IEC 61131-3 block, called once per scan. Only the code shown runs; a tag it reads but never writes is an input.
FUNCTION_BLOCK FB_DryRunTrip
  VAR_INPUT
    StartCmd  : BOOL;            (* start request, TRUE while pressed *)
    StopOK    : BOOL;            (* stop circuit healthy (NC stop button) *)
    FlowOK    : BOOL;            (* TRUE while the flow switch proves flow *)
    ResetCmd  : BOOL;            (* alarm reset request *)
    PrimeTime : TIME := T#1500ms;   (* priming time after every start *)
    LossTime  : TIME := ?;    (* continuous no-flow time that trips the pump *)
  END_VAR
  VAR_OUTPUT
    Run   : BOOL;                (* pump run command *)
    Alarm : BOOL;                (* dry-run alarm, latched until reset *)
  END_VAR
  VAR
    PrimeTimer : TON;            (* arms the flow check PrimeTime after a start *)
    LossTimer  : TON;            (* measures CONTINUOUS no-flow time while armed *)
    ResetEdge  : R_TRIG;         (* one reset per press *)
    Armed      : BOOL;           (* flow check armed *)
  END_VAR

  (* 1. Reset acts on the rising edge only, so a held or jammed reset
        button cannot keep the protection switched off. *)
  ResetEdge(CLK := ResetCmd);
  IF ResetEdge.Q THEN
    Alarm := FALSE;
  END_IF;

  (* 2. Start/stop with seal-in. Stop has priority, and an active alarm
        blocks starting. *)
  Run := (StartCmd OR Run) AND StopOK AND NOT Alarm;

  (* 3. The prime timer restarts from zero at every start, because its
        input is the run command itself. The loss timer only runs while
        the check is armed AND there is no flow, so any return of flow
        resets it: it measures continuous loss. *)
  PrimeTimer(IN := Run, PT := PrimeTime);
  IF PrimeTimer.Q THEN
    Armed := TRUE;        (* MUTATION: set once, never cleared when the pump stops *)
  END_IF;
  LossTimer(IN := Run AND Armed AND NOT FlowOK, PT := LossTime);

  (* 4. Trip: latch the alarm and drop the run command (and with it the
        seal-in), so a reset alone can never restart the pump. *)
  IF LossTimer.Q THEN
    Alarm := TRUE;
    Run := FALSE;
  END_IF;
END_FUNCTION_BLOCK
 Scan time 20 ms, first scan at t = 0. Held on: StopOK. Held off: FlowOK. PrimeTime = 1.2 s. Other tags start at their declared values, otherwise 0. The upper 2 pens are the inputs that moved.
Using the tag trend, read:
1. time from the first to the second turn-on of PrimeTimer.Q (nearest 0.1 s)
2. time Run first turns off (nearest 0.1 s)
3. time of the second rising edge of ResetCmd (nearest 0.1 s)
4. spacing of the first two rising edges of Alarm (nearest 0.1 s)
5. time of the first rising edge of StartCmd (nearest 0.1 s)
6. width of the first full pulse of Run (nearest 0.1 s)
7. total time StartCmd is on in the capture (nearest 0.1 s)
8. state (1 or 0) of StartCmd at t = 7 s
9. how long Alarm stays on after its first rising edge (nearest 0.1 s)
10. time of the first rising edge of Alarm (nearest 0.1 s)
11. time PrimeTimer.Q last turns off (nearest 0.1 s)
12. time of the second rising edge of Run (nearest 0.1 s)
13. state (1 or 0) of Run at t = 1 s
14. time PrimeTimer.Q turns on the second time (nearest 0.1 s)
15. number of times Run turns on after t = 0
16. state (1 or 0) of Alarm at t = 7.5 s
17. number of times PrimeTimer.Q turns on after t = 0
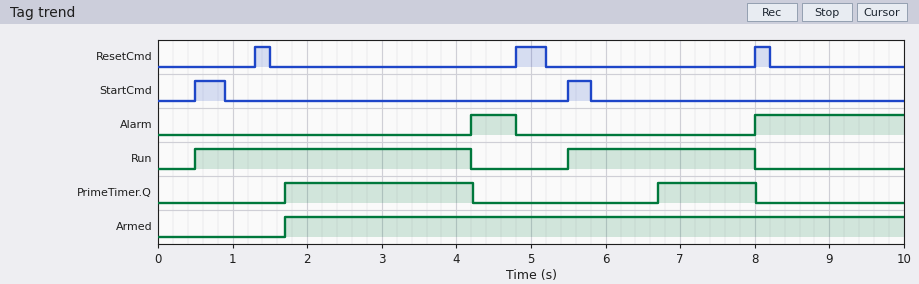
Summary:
5.0 s
4.2 s
4.8 s
3.8 s
0.5 s
3.7 s
0.7 s
0
0.6 s
4.2 s
8.0 s
5.5 s
1
6.7 s
2
0
2
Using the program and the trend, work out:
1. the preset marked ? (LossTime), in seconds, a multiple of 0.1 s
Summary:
2.5 s
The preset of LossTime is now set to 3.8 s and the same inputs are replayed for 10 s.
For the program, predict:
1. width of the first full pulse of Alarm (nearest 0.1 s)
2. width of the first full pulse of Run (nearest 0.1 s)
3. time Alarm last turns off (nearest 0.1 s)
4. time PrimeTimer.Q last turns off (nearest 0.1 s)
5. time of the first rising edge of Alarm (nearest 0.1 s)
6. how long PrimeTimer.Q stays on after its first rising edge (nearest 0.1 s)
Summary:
2.5 s
5.0 s
8.0 s
5.5 s
5.5 s
3.8 s
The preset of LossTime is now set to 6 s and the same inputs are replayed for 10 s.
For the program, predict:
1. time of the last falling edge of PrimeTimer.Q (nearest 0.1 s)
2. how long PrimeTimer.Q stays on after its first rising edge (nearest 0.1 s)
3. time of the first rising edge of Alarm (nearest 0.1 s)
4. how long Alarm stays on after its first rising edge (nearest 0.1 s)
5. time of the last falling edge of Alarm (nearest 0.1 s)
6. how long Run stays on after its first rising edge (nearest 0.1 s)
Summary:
7.7 s
6.0 s
7.7 s
0.3 s
8.0 s
7.2 s
